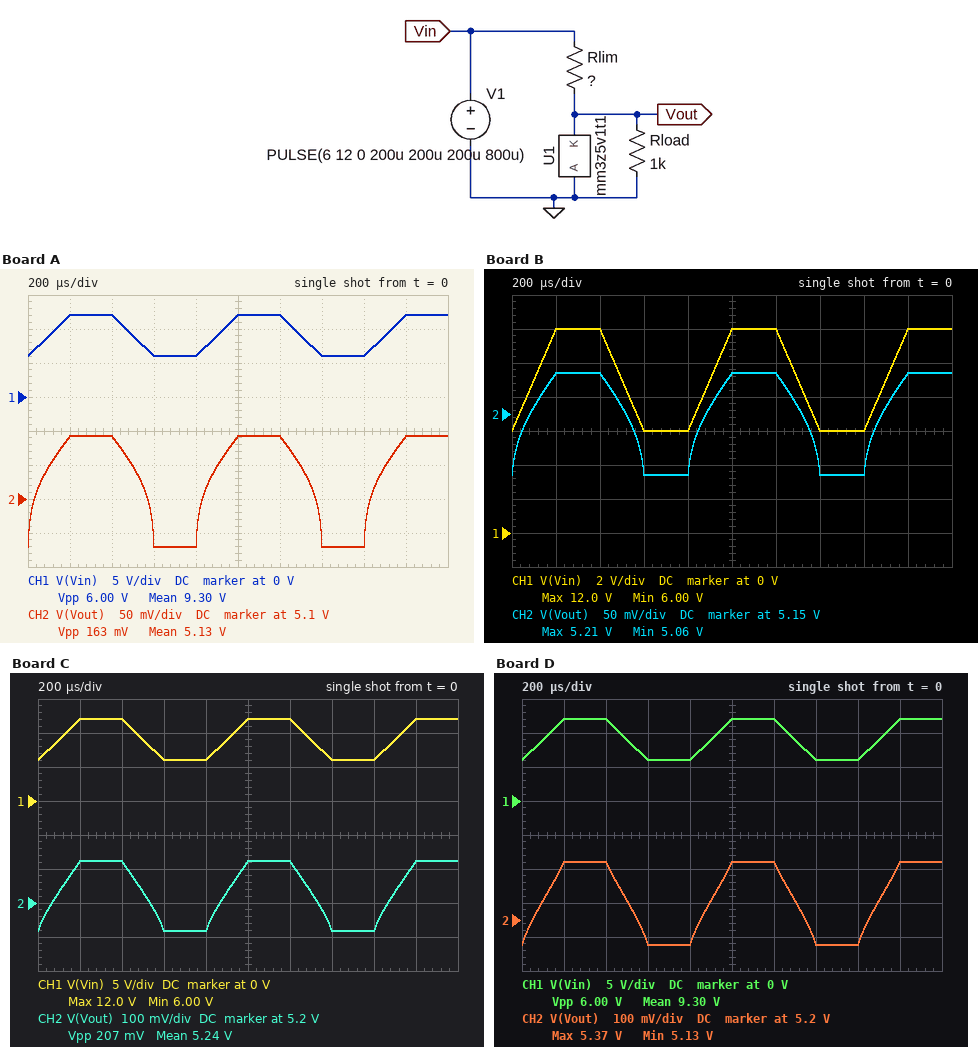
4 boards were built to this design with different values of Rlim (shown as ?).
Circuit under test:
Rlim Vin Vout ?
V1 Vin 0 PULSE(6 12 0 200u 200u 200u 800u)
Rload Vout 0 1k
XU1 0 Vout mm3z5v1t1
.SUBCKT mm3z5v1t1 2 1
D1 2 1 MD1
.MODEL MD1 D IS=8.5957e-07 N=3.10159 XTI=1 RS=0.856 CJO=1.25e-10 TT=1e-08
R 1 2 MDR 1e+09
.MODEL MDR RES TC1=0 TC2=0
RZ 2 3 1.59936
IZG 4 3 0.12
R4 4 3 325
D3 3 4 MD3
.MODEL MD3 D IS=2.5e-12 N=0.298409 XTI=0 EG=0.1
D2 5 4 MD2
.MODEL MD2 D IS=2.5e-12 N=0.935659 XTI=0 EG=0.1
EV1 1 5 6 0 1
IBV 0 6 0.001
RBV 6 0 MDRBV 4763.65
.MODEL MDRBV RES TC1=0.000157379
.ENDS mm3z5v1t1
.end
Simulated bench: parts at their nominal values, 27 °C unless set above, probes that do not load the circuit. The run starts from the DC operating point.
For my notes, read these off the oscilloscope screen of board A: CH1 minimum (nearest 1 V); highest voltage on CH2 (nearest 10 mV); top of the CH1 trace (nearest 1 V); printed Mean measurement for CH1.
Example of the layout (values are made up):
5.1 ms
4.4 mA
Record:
6 V
5.19 V
12 V
9.30 V
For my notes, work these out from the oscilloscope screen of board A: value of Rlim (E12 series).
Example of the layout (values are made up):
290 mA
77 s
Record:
180 Ω
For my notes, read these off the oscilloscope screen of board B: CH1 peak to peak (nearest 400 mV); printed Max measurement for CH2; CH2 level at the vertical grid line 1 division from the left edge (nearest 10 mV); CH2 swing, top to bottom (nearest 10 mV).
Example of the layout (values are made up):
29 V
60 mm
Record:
6.0 V
5.21 V
5.21 V
150 mV
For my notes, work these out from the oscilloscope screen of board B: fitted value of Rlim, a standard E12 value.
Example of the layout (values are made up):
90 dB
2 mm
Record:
150 Ω
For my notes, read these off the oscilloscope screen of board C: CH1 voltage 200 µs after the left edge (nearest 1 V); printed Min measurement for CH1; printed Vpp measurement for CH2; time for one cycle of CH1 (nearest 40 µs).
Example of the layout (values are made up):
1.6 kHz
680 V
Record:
12 V
6.00 V
207 mV
800 µs
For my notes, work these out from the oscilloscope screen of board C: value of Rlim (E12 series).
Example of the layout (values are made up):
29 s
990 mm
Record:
68 Ω
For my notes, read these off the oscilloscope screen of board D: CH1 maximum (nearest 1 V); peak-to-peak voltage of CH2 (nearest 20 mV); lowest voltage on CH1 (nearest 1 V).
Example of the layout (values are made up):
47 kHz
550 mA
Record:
12 V
240 mV
6 V
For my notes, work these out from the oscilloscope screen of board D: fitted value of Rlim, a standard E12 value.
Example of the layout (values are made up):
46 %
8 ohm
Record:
56 Ω
